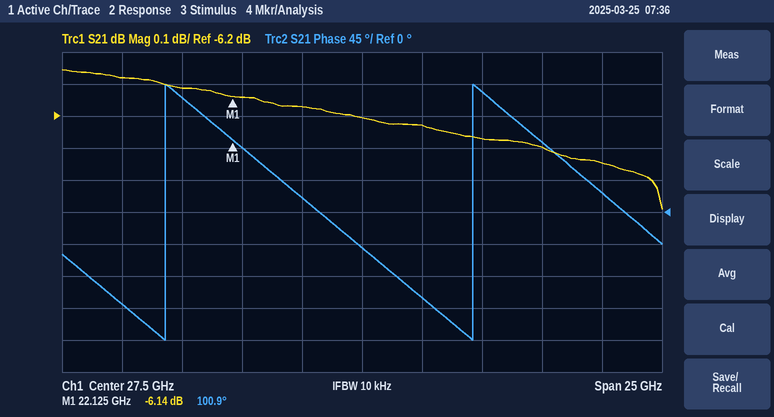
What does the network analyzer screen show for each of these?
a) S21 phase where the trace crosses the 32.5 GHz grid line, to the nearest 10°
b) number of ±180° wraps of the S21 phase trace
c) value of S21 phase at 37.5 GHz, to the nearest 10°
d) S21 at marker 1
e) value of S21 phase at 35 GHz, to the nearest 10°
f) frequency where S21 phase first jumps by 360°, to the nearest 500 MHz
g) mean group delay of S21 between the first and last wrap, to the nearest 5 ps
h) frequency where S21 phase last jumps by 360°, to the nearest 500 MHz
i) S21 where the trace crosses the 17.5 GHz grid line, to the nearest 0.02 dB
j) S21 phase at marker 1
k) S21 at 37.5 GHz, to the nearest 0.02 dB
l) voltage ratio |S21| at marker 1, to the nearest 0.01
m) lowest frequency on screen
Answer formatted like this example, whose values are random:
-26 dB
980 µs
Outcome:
170°
2
30°
-6.14 dB
100°
19.5 GHz
80 ps
32.0 GHz
-6.08 dB
100.9°
-6.34 dB
0.49
15 GHz
